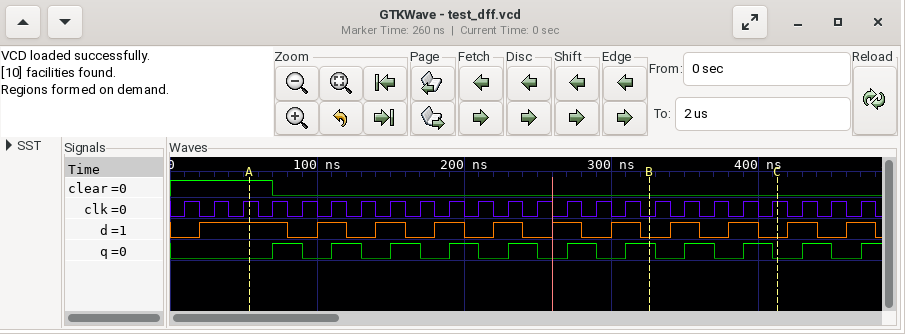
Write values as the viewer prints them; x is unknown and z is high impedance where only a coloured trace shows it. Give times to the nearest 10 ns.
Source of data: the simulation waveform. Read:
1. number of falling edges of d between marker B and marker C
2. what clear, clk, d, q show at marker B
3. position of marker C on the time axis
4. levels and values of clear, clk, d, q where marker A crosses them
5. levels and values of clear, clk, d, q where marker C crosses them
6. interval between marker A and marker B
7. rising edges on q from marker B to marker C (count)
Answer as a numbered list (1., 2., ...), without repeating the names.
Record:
1. 2
2. clear=0, clk=0, d=0, q=1
3. 410 ns
4. clear=1, clk=1, d=1, q=0
5. clear=0, clk=1, d=0, q=0
6. 270 ns
7. 2
